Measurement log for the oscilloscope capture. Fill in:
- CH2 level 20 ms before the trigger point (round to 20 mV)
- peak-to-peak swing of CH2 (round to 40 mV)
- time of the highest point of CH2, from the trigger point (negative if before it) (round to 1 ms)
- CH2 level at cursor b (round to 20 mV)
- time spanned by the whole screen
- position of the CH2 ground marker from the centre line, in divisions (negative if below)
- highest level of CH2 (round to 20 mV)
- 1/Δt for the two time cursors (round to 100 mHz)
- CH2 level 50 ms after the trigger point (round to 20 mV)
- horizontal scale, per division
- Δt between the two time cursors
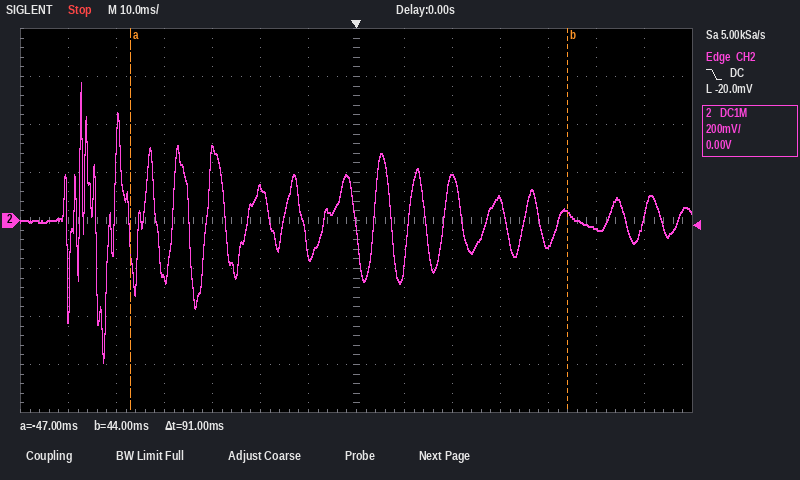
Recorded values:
140 mV
1.16 V
-57 ms
40 mV
140 ms
0.0 div
580 mV
11.0 Hz
-40 mV
10 ms
91 ms
